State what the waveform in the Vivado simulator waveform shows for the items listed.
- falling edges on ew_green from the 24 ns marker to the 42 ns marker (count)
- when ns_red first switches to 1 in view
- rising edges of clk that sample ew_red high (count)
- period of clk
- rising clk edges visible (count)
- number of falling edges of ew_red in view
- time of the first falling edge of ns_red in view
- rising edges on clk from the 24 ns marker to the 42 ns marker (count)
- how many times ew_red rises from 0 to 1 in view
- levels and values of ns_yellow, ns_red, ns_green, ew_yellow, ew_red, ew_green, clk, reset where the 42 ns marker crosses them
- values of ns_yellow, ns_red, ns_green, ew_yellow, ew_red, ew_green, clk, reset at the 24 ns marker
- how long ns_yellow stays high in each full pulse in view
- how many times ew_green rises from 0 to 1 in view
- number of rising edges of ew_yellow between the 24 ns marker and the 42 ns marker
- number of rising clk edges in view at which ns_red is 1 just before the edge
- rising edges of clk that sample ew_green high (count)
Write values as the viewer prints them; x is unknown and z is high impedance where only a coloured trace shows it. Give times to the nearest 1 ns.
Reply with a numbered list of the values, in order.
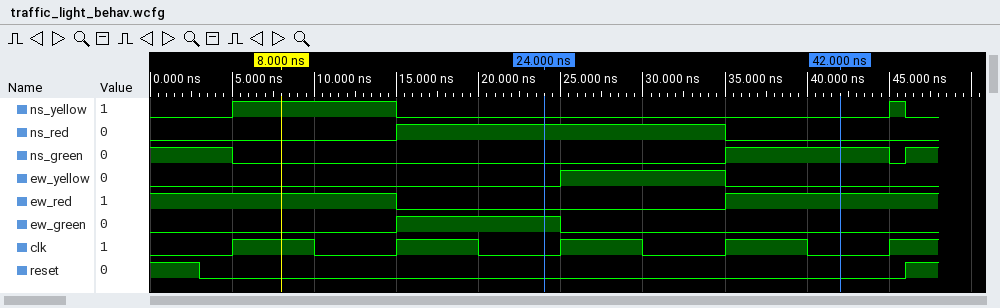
1. 1
2. 15 ns
3. 3
4. 10 ns
5. 5
6. 1
7. 35 ns
8. 2
9. 1
10. ns_yellow=0, ns_red=0, ns_green=1, ew_yellow=0, ew_red=1, ew_green=0, clk=0, reset=0
11. ns_yellow=0, ns_red=1, ns_green=0, ew_yellow=0, ew_red=0, ew_green=1, clk=0, reset=0
12. 10 ns, 1 ns
13. 1
14. 1
15. 2
16. 1
